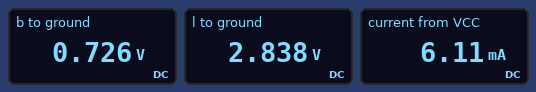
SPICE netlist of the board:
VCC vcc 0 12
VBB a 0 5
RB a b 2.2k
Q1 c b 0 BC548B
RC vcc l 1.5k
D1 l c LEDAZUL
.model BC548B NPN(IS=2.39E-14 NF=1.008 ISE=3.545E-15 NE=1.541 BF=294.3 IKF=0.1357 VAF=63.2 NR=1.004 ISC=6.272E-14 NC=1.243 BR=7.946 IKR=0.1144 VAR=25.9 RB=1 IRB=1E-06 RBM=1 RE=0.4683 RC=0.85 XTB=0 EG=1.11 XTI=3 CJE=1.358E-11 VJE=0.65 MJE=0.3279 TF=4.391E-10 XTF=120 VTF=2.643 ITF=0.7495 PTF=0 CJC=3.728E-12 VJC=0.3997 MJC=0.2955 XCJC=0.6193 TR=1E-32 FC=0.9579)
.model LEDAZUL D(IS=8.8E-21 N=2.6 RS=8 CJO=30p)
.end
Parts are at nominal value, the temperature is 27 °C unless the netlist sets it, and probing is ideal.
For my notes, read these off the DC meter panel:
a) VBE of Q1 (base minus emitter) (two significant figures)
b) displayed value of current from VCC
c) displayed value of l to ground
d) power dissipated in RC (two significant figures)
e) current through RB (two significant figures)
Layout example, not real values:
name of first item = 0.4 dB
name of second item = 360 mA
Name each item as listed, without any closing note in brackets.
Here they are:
VBE of Q1 (base minus emitter) = 730 mV
displayed value of current from VCC = 6.11 mA
displayed value of l to ground = 2.838 V
power dissipated in RC = 56 mW
current through RB = 1.9 mA
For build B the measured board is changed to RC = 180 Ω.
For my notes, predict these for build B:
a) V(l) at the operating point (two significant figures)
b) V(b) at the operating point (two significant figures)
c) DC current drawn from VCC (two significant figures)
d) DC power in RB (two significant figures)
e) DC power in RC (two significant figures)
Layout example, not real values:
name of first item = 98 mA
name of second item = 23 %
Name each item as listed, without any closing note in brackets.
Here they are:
V(l) at the operating point = 3.4 V
V(b) at the operating point = 780 mV
DC current drawn from VCC = 48 mA
DC power in RB = 8.1 mW
DC power in RC = 410 mW
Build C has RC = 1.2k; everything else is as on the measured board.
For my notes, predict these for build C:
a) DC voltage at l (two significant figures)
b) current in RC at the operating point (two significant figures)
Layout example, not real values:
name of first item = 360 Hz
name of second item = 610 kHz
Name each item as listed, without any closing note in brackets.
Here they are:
DC voltage at l = 2.9 V
current in RC at the operating point = 7.6 mA
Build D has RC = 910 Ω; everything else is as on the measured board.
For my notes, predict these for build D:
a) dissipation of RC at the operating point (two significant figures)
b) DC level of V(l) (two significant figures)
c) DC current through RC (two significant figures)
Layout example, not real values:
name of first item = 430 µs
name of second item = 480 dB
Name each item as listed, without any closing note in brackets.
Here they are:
dissipation of RC at the operating point = 91 mW
DC level of V(l) = 2.9 V
DC current through RC = 10 mA
